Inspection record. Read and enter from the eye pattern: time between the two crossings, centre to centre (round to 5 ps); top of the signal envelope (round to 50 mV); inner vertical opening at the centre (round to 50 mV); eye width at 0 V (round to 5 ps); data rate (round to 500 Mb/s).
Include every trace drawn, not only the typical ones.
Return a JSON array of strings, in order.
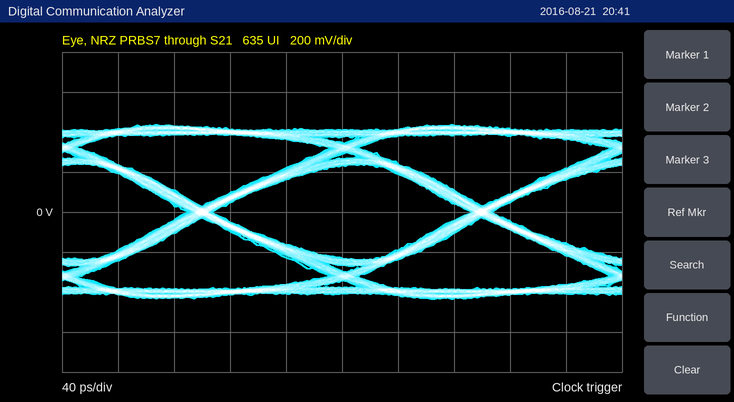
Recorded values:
["200 ps", "450 mV", "450 mV", "185 ps", "5.0 Gb/s"]
